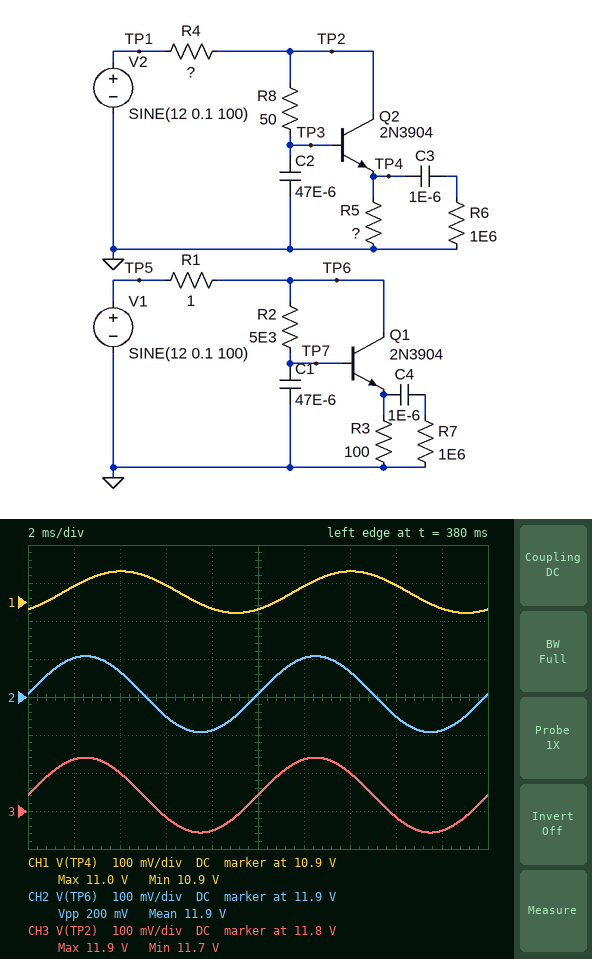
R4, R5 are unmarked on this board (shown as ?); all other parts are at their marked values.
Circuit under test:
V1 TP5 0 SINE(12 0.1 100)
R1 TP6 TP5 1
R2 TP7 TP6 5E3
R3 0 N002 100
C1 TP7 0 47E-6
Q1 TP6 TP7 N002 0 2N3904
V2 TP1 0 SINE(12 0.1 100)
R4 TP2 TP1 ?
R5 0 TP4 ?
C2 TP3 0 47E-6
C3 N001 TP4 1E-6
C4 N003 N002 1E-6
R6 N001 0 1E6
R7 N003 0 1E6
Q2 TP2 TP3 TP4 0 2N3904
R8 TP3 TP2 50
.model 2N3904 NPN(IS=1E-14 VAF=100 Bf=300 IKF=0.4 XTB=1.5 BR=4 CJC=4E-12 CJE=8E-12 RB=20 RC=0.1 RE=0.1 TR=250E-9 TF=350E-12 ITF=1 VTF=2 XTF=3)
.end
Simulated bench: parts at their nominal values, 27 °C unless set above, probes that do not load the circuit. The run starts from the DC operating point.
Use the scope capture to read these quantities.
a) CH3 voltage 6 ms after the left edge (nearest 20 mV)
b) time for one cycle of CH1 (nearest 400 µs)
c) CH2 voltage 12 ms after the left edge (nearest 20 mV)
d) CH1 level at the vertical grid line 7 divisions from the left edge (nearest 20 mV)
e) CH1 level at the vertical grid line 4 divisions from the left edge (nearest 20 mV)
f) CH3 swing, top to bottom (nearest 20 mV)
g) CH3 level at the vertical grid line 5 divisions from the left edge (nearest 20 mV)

11.78 V
10.0 ms
12.00 V
10.98 V
10.88 V
200 mV
11.84 V
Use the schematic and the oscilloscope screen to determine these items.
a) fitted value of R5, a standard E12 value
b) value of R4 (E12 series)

47 Ω
0.68 Ω
